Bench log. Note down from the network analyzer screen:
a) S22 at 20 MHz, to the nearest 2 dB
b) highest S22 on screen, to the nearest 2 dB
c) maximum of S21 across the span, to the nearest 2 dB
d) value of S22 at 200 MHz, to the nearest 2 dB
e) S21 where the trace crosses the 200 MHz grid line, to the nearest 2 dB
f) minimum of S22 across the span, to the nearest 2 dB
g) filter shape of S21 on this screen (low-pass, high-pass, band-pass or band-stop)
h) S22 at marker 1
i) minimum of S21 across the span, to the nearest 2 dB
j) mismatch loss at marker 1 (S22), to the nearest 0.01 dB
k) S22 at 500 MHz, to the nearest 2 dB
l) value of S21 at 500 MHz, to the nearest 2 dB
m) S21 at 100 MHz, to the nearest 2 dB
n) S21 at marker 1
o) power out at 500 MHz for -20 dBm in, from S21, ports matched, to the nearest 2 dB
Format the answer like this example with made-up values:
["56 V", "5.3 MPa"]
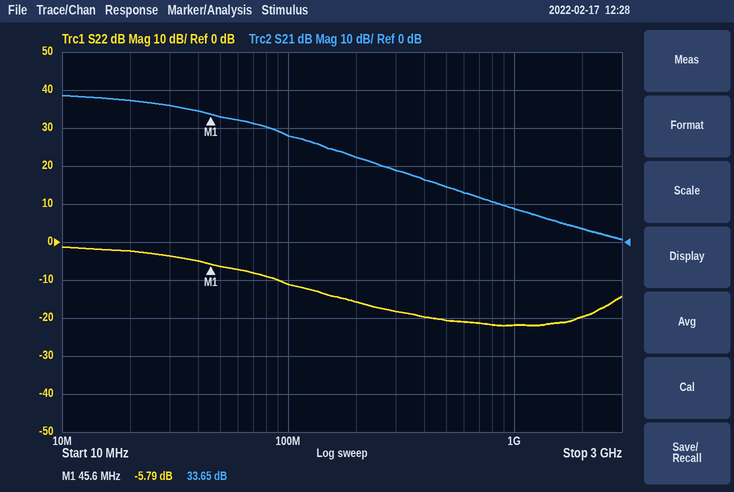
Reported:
["-2 dB", "-2 dB", "38 dB", "-16 dB", "22 dB", "-22 dB", "low-pass", "-5.79 dB", "0 dB", "1.33 dB", "-20 dB", "14 dB", "28 dB", "33.65 dB", "-6 dBm"]
